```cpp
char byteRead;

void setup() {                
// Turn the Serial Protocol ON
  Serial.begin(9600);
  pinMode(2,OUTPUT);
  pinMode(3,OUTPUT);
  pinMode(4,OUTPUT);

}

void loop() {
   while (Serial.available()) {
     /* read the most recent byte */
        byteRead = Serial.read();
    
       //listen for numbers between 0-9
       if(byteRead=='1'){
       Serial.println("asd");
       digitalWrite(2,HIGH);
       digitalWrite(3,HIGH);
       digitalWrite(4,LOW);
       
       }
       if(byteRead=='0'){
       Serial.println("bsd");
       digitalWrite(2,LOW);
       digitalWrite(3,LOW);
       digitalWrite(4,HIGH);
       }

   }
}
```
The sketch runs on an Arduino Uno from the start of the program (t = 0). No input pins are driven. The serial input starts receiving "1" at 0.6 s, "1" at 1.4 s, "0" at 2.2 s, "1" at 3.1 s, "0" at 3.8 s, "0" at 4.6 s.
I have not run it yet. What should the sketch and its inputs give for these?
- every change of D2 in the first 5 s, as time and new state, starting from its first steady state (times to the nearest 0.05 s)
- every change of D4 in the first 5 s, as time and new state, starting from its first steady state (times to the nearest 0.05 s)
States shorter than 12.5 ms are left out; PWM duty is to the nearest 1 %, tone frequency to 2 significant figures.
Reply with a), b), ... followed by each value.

a) 0 s low; 0.6 s high; 2.2 s low; 3.1 s high; 3.8 s low
b) 0 s low; 2.2 s high; 3.1 s low; 3.8 s high
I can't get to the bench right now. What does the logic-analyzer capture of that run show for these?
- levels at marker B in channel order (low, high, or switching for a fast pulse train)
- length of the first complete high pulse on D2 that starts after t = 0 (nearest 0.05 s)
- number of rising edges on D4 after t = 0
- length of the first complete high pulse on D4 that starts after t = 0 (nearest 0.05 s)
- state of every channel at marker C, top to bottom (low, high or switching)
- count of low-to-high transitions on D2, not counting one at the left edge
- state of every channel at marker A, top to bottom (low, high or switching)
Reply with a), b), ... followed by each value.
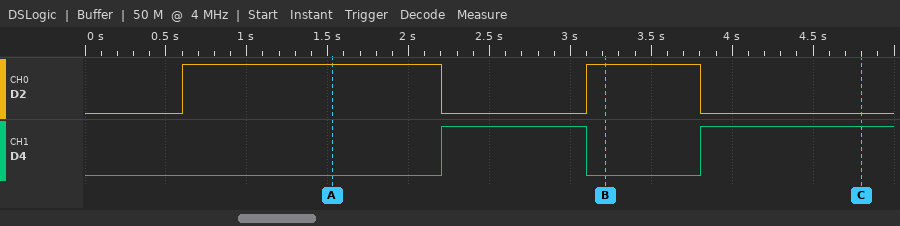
a) D2 high, D4 low
b) 1.60 s
c) 2
d) 0.90 s
e) D2 low, D4 high
f) 2
g) D2 high, D4 low
